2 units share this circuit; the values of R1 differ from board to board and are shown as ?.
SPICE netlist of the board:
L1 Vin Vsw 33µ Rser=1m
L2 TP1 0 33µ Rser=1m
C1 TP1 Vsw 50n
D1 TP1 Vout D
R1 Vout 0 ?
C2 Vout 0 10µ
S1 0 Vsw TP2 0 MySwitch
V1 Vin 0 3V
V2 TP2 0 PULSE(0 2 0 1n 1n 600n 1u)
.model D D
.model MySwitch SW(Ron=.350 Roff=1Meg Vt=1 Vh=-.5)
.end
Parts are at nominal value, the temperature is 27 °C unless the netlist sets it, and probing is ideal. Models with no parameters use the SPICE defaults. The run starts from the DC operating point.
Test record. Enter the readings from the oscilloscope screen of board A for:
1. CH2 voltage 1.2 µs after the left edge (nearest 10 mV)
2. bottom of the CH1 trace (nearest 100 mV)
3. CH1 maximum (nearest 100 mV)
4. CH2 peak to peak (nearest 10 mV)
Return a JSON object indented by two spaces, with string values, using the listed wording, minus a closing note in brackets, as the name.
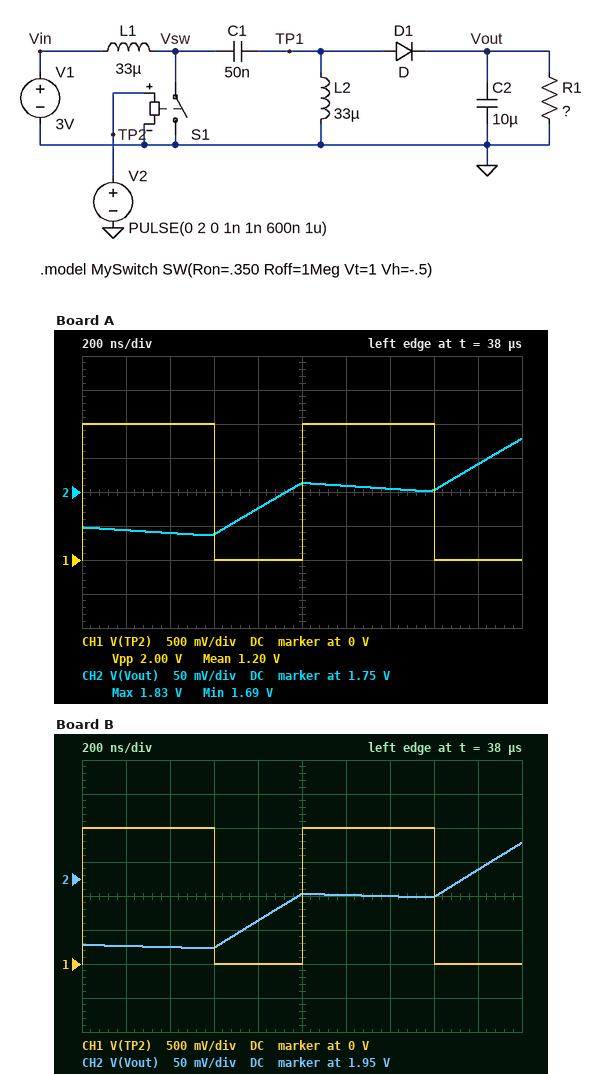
{
  "CH2 voltage 1.2 µs after the left edge": "1.76 V",
  "bottom of the CH1 trace": "0 V",
  "CH1 maximum": "2.0 V",
  "CH2 peak to peak": "140 mV"
}
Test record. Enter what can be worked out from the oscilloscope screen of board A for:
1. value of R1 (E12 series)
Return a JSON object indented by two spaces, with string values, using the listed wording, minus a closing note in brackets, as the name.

{
  "value of R1": "8.2 Ω"
}
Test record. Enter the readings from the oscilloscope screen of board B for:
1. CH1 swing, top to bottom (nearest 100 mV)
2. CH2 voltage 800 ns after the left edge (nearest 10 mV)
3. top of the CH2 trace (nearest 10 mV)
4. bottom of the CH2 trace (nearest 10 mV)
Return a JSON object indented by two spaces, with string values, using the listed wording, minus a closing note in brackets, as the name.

{
  "CH1 swing, top to bottom": "2.0 V",
  "CH2 voltage 800 ns after the left edge": "1.89 V",
  "top of the CH2 trace": "2.00 V",
  "bottom of the CH2 trace": "1.85 V"
}
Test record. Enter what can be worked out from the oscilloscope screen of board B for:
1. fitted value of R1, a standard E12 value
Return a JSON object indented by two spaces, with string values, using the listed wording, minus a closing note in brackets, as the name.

{
  "fitted value of R1, a standard E12 value": "22 Ω"
}
